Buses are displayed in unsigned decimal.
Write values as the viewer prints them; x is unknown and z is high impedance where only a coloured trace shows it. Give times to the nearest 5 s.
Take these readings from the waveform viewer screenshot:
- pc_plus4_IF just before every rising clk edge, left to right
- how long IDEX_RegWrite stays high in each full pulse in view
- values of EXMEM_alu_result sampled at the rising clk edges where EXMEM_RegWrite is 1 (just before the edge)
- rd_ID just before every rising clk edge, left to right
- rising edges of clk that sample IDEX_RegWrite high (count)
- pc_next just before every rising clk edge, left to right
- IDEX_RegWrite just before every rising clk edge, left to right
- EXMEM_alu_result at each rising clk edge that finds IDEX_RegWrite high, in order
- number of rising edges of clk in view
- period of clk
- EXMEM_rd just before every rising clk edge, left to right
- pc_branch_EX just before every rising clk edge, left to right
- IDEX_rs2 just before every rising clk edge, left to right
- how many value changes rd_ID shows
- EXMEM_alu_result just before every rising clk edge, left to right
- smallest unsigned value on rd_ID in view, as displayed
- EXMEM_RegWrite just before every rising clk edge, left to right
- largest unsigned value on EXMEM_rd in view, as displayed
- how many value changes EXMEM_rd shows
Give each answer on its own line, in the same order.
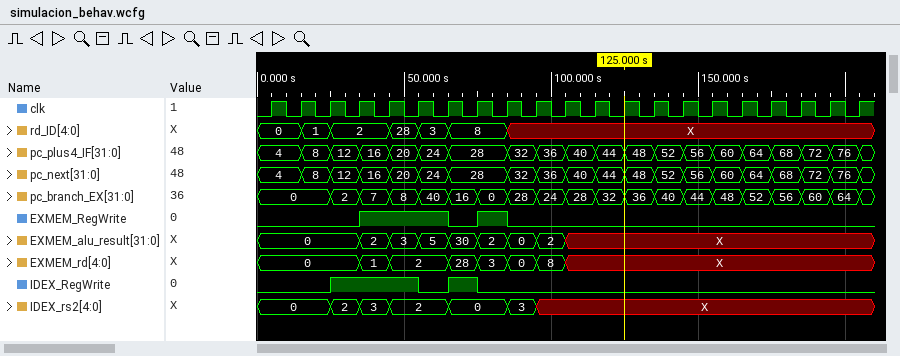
4, 4, 8, 12, 16, 20, 24, 28, 28, 32, 36, 40, 44, 48, 52, 56, 60, 64, 68, 72, 76
30 s, 10 s
2, 3, 5, 2
0, 0, 1, 2, 2, 28, 3, 8, 8, X, X, X, X, X, X, X, X, X, X, X, X
4
4, 4, 8, 12, 16, 20, 24, 28, 28, 32, 36, 40, 44, 48, 52, 56, 60, 64, 68, 72, 76
0 0 0 1 1 1 0 1 0 0 0 0 0 0 0 0 0 0 0 0 0
0, 2, 3, 30
21
10 s
0, 0, 0, 0, 1, 2, 2, 28, 3, 0, 8, X, X, X, X, X, X, X, X, X, X
0, 0, 0, 2, 7, 8, 40, 16, 0, 28, 24, 28, 32, 36, 40, 44, 48, 52, 56, 60, 64
0, 0, 0, 2, 3, 2, 2, 0, 0, 3, X, X, X, X, X, X, X, X, X, X, X
6
0, 0, 0, 0, 2, 3, 5, 30, 2, 0, 2, X, X, X, X, X, X, X, X, X, X
0
0 0 0 0 1 1 1 0 1 0 0 0 0 0 0 0 0 0 0 0 0
28
7
